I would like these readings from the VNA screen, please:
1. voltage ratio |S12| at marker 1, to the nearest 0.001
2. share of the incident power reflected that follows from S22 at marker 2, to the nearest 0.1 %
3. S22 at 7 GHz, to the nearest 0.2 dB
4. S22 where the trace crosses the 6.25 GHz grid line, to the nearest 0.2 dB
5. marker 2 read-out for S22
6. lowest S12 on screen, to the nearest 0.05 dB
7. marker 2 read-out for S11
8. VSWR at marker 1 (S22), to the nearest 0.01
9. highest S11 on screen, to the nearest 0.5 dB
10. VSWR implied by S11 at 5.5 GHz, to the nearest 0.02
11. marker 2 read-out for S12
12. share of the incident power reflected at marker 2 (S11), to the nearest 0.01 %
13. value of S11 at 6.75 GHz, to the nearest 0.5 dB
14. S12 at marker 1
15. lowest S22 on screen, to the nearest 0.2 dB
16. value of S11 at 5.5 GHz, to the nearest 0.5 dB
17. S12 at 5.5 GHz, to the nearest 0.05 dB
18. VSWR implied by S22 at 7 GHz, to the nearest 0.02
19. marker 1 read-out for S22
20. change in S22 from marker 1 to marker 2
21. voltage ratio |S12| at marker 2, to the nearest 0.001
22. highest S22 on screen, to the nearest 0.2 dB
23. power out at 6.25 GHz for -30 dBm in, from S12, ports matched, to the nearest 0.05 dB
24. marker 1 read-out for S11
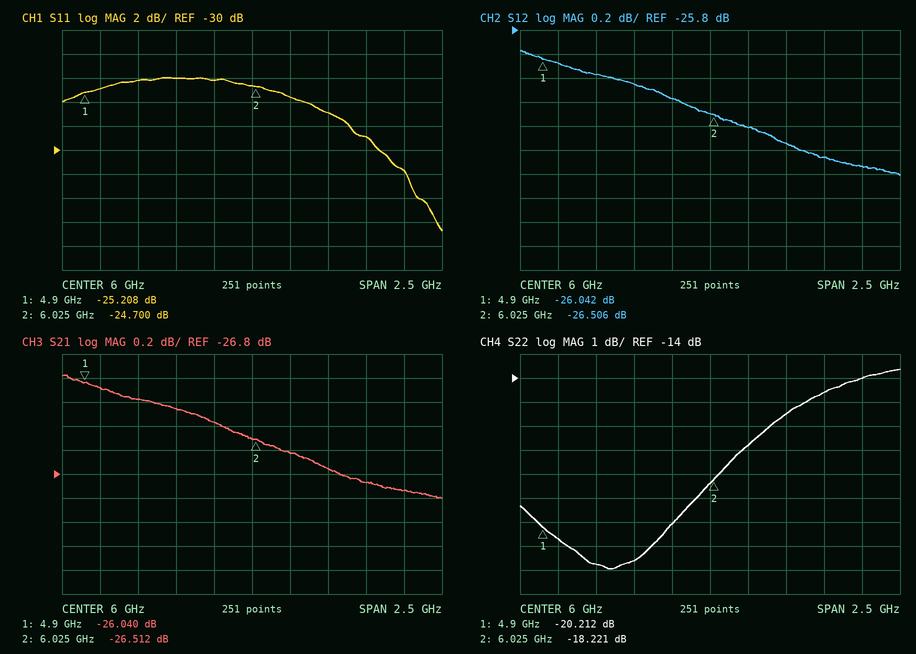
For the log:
0.050
1.5 %
-14.0 dB
-16.8 dB
-18.221 dB
-27.00 dB
-24.700 dB
1.22
-24.0 dB
1.14
-26.506 dB
0.34 %
-29.0 dB
-26.042 dB
-22.0 dB
-24.0 dB
-26.25 dB
1.50
-20.212 dB
1.991 dB
0.047
-13.6 dB
-56.60 dBm
-25.208 dB
